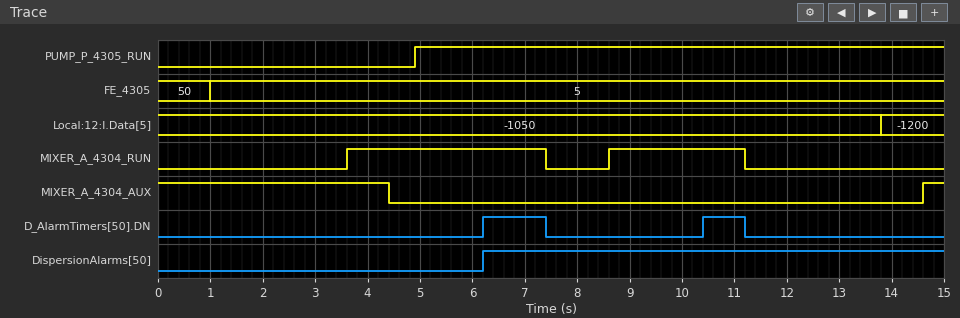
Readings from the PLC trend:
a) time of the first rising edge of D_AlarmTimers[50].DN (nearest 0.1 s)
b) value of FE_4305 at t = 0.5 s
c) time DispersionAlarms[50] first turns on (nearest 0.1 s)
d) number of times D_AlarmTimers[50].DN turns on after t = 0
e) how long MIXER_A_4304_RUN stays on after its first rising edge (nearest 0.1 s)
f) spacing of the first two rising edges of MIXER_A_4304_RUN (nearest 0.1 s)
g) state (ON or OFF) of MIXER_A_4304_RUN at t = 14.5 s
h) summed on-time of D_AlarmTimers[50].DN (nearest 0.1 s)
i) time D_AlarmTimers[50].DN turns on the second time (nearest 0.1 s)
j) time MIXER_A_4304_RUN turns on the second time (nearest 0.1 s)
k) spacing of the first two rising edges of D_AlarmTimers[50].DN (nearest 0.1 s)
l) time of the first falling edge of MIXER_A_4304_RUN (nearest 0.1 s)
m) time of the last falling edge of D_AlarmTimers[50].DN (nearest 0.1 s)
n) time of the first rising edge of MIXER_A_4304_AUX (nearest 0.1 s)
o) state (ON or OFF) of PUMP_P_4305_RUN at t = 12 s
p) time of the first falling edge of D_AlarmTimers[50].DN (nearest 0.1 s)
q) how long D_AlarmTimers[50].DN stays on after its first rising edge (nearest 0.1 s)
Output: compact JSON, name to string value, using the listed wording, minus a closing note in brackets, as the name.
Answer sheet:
{"time of the first rising edge of D_AlarmTimers[50].DN": "6.2 s", "value of FE_4305 at t = 0.5 s": "50", "time DispersionAlarms[50] first turns on": "6.2 s", "number of times D_AlarmTimers[50].DN turns on after t = 0": "2", "how long MIXER_A_4304_RUN stays on after its first rising edge": "3.8 s", "spacing of the first two rising edges of MIXER_A_4304_RUN": "5.0 s", "state (ON or OFF) of MIXER_A_4304_RUN at t = 14.5 s": "OFF", "summed on-time of D_AlarmTimers[50].DN": "2.0 s", "time D_AlarmTimers[50].DN turns on the second time": "10.4 s", "time MIXER_A_4304_RUN turns on the second time": "8.6 s", "spacing of the first two rising edges of D_AlarmTimers[50].DN": "4.2 s", "time of the first falling edge of MIXER_A_4304_RUN": "7.4 s", "time of the last falling edge of D_AlarmTimers[50].DN": "11.2 s", "time of the first rising edge of MIXER_A_4304_AUX": "14.6 s", "state (ON or OFF) of PUMP_P_4305_RUN at t = 12 s": "ON", "time of the first falling edge of D_AlarmTimers[50].DN": "7.4 s", "how long D_AlarmTimers[50].DN stays on after its first rising edge": "1.2 s"}
